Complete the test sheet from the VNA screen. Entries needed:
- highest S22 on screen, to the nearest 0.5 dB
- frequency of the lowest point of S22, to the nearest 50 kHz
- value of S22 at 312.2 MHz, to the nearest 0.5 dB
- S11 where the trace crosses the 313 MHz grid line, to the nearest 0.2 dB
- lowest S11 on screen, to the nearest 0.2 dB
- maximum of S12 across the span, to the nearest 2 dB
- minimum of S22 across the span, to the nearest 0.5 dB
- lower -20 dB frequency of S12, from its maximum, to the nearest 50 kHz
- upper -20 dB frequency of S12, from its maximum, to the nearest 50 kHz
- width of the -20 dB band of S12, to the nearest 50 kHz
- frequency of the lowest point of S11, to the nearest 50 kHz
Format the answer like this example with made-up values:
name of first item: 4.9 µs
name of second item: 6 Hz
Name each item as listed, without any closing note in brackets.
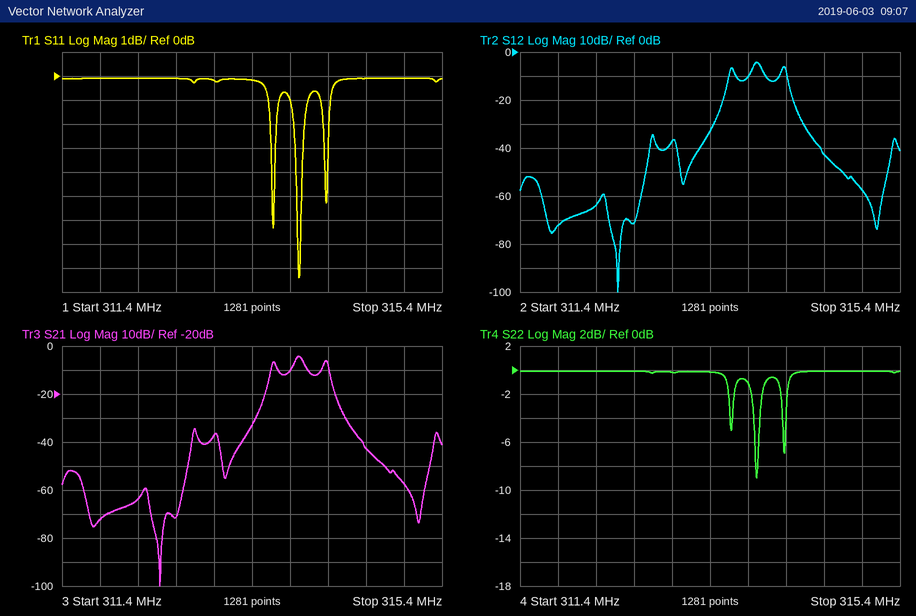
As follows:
highest S22 on screen, to the nearest 0.5 dB: 0.0 dB
frequency of the lowest point of S22, to the nearest 50 kHz: 313.90 MHz
value of S22 at 312.2 MHz, to the nearest 0.5 dB: 0.0 dB
S11 where the trace crosses the 313 MHz grid line, to the nearest 0.2 dB: -0.2 dB
lowest S11 on screen, to the nearest 0.2 dB: -8.4 dB
maximum of S12 across the span, to the nearest 2 dB: -4 dB
minimum of S22 across the span, to the nearest 0.5 dB: -9.0 dB
lower -20 dB frequency of S12, from its maximum, to the nearest 50 kHz: 313.50 MHz
upper -20 dB frequency of S12, from its maximum, to the nearest 50 kHz: 314.30 MHz
width of the -20 dB band of S12, to the nearest 50 kHz: 800 kHz
frequency of the lowest point of S11, to the nearest 50 kHz: 313.90 MHz
